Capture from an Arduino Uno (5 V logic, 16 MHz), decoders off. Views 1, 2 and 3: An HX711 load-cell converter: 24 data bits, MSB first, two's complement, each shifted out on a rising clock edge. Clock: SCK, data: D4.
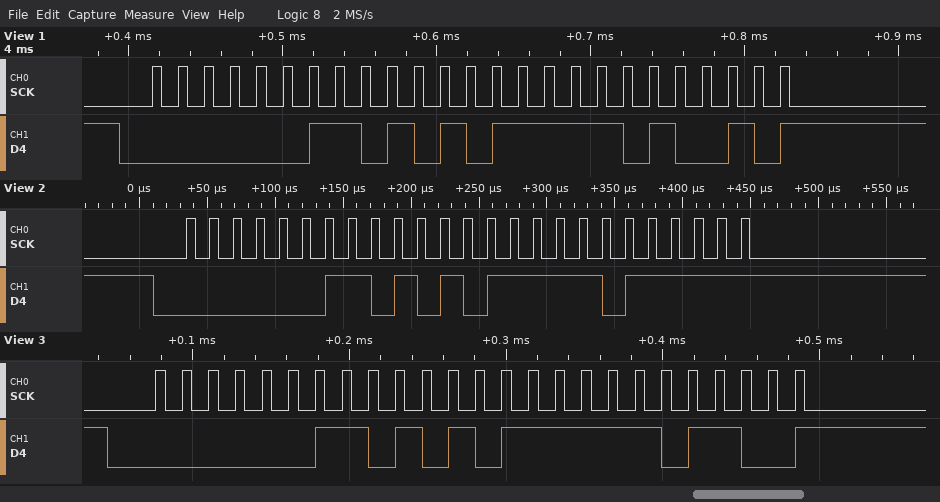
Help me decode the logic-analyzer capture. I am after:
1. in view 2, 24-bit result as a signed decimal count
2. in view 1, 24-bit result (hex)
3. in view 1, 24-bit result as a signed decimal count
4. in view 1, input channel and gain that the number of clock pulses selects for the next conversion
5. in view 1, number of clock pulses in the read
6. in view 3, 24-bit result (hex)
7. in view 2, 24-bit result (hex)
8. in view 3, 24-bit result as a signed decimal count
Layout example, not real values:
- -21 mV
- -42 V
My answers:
- 219103
- 0x0357D2
- 219090
- channel A, gain 128
- 25
- 0x0357EC
- 0x0357DF
- 219116
